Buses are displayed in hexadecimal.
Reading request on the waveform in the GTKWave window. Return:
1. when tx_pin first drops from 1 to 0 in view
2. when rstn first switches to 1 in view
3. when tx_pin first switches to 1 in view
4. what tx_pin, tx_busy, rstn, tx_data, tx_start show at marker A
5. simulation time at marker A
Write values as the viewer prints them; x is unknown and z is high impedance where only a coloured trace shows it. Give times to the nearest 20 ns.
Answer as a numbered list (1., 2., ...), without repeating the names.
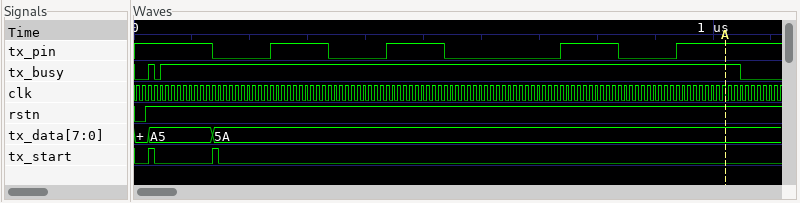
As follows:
1. 140 ns
2. 20 ns
3. 240 ns
4. tx_pin=1, tx_busy=1, rstn=1, tx_data=5A, tx_start=0
5. 1020 ns
